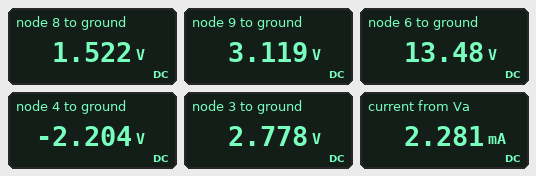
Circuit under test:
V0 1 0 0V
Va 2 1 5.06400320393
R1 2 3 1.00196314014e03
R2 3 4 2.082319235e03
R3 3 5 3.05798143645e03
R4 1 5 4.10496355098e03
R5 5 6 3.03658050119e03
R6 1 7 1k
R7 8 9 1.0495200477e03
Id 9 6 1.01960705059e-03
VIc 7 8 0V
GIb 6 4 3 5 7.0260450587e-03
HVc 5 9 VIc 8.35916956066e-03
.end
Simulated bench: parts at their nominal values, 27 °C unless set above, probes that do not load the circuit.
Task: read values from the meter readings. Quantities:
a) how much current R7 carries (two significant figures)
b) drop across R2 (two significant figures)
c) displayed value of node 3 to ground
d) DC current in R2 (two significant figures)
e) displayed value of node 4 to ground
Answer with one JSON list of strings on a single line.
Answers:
["1.5 mA", "5.0 V", "2.778 V", "2.4 mA", "-2.204 V"]
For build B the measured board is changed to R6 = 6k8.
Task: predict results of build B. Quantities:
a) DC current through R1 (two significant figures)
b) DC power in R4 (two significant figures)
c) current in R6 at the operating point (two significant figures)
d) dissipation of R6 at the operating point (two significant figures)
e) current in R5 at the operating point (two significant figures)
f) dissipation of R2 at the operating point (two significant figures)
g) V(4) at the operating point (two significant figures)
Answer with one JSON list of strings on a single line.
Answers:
["1.4 mA", "3.6 mW", "490 µA", "1.6 mW", "2.5 mA", "4.7 mW", "520 mV"]
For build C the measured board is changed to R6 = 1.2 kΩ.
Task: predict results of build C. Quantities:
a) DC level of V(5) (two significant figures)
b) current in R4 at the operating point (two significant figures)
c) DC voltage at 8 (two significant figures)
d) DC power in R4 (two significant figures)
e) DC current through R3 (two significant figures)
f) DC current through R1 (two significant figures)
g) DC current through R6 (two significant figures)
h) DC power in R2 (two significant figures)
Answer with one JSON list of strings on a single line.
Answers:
["3.2 V", "780 µA", "1.7 V", "2.5 mW", "110 µA", "2.2 mA", "1.4 mA", "11 mW"]
